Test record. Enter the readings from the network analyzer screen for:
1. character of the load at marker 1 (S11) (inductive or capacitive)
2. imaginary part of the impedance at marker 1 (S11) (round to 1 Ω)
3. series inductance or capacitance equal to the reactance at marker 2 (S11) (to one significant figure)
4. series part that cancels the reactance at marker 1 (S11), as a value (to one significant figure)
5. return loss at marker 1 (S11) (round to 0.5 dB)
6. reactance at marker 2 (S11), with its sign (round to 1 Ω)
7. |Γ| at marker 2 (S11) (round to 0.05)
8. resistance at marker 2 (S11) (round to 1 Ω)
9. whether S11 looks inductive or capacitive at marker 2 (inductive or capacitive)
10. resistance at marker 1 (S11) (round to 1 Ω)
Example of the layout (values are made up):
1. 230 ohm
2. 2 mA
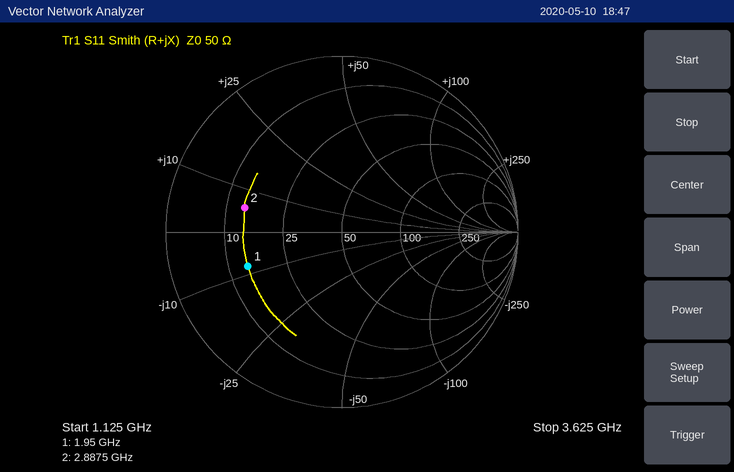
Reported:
1. capacitive
2. -8 Ω
3. 300 pH
4. 700 pH
5. 5.0 dB
6. +6 Ω
7. 0.55
8. 14 Ω
9. inductive
10. 14 Ω
